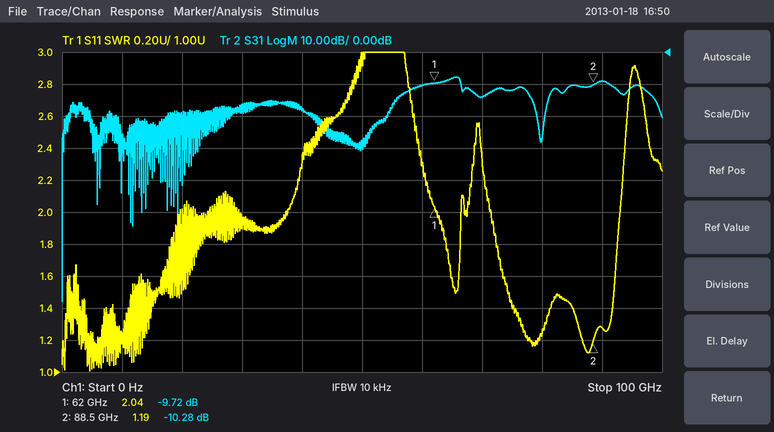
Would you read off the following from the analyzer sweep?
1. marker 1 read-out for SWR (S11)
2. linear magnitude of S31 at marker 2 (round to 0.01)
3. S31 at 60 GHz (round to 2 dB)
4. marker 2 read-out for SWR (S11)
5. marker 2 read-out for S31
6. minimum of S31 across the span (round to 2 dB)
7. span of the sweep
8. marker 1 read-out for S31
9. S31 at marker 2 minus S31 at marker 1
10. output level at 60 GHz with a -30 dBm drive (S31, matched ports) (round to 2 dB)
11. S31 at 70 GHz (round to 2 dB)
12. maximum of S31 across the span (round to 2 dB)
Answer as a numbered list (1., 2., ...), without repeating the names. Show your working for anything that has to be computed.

1. 2.04
2. 10^(-10.28/20) ≈ 0.31
3. -10 dB
4. 1.19
5. -10.28 dB
6. -78 dB
7. 100 GHz
8. -9.72 dB
9. -10.28 − (-9.72) = -0.56 dB
10. -30 dBm + (-10 dB) = -40 dBm
11. -14 dB
12. -8 dB
